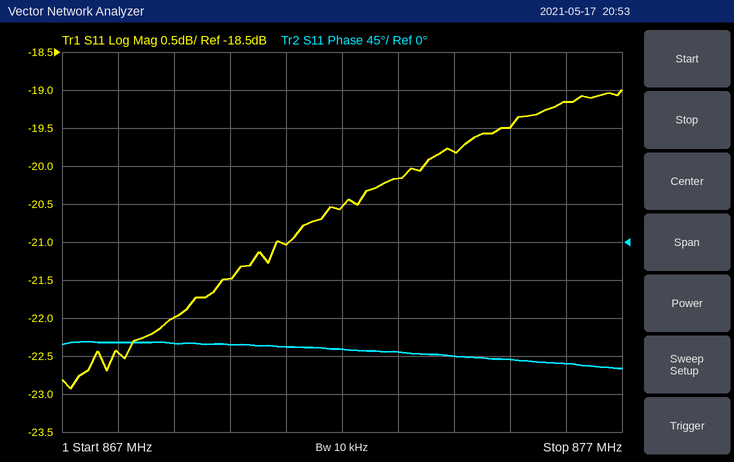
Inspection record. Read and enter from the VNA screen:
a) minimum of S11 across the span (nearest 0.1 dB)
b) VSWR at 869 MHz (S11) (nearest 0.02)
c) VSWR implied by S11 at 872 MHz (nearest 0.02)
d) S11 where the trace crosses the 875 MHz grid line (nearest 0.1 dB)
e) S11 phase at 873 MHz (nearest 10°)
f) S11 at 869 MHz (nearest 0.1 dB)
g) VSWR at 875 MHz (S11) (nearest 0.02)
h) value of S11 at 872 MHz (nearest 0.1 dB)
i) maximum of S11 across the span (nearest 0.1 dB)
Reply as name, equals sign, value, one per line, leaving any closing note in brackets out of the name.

minimum of S11 across the span = -22.9 dB
VSWR at 869 MHz (S11) = 1.18
VSWR implied by S11 at 872 MHz = 1.20
S11 where the trace crosses the 875 MHz grid line = -19.5 dB
S11 phase at 873 MHz = -130°
S11 at 869 MHz = -22.0 dB
VSWR at 875 MHz (S11) = 1.24
value of S11 at 872 MHz = -20.5 dB
maximum of S11 across the span = -19.0 dB
